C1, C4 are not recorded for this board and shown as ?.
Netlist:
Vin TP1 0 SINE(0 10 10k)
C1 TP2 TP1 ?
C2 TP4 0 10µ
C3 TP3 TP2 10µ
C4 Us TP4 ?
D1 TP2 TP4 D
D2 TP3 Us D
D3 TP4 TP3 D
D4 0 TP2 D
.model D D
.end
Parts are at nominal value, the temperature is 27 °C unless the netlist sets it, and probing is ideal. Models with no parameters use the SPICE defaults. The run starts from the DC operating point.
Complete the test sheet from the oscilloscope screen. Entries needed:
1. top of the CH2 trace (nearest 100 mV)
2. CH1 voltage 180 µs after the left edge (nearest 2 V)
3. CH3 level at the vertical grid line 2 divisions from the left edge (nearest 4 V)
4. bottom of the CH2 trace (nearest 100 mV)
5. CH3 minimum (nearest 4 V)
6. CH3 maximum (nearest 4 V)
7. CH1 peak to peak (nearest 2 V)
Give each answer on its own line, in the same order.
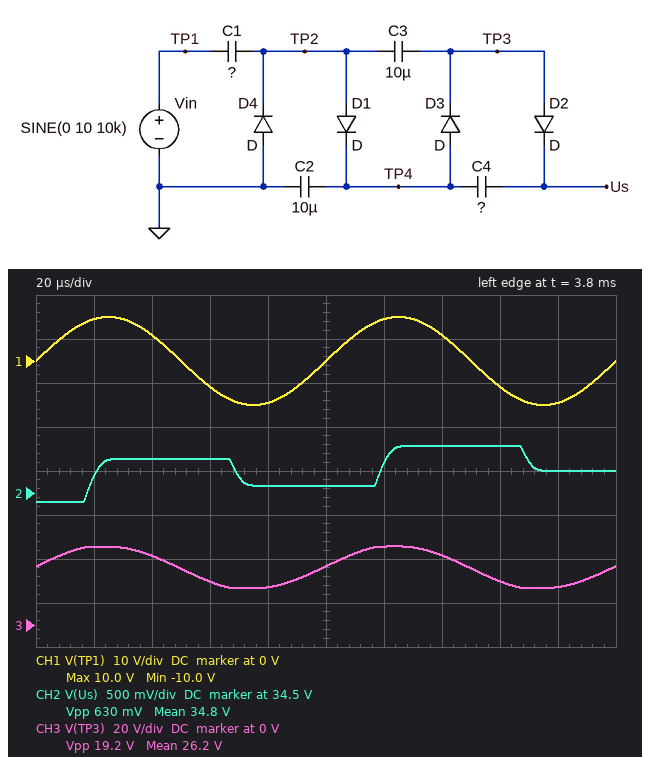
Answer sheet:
35.0 V
-10 V
32 V
34.4 V
16 V
36 V
20 V
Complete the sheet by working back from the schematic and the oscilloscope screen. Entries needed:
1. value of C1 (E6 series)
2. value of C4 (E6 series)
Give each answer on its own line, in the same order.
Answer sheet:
4.7 µF
22 µF
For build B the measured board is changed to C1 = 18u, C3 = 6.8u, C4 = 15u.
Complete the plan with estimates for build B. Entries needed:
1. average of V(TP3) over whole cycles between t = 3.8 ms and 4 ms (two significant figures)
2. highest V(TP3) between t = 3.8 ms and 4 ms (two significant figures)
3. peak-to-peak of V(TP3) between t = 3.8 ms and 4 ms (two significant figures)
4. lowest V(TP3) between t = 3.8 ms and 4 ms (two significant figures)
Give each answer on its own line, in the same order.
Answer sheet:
28 V
38 V
20 V
18 V
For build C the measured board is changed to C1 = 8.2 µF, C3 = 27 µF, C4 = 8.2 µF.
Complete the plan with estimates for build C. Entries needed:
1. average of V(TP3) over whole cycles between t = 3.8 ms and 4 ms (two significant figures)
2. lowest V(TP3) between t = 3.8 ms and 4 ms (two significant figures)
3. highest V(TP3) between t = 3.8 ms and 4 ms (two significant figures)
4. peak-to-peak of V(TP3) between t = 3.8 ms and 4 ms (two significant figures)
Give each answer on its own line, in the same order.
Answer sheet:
27 V
17 V
37 V
20 V
